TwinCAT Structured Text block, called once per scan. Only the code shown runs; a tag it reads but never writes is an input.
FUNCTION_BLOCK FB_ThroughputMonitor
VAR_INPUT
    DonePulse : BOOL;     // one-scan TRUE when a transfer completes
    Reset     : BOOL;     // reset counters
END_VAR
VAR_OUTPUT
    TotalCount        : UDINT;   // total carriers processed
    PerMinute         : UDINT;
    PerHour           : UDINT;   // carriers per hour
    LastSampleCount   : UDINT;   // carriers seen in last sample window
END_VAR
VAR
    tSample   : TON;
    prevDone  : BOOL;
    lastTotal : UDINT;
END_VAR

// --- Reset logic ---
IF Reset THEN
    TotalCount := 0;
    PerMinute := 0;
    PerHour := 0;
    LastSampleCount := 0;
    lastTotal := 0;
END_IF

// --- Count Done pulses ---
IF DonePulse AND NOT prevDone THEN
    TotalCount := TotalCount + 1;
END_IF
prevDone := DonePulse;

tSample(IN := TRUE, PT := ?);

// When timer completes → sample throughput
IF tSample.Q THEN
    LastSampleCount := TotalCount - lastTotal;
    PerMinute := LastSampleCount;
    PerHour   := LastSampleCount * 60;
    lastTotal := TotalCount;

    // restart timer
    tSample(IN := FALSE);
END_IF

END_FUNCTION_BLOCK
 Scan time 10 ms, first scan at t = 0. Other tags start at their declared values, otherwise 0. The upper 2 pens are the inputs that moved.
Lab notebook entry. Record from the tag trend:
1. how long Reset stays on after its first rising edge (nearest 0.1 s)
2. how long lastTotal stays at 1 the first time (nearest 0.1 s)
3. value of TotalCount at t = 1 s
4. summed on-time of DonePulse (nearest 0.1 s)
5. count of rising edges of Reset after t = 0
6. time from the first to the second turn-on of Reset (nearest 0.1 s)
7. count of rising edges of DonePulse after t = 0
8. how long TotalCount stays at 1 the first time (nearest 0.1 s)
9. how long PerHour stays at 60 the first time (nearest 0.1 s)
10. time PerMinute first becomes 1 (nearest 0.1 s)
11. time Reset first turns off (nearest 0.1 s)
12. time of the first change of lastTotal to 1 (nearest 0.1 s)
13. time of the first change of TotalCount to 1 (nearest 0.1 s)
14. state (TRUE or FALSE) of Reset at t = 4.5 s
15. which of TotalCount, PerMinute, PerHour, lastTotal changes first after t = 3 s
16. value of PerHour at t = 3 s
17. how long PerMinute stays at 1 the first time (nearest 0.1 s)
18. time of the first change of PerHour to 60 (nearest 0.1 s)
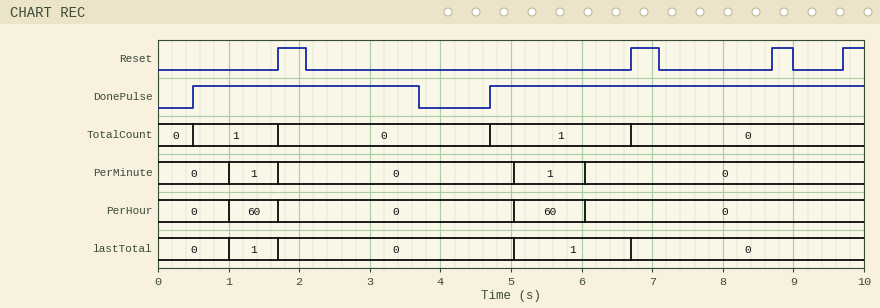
0.4 s
0.7 s
1
8.5 s
4
5.0 s
2
1.2 s
0.7 s
1.0 s
2.1 s
1.0 s
0.5 s
FALSE
TotalCount
0
0.7 s
1.0 s
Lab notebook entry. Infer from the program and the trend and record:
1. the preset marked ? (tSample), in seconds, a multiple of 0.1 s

1.0 s
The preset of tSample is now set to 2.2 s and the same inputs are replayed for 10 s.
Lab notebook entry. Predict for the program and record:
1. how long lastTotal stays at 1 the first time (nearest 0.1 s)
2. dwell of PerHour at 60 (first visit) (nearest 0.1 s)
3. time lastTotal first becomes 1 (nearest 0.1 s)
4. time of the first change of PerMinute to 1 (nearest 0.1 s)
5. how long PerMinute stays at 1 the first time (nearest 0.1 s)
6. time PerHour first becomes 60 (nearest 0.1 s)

0.1 s
0.1 s
6.6 s
6.6 s
0.1 s
6.6 s
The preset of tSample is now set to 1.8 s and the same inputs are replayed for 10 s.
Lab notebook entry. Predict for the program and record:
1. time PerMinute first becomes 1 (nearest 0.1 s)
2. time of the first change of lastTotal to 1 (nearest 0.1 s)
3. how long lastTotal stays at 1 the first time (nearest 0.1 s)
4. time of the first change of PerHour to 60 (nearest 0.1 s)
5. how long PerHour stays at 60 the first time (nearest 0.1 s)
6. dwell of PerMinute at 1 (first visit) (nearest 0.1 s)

5.4 s
5.4 s
1.3 s
5.4 s
1.3 s
1.3 s
